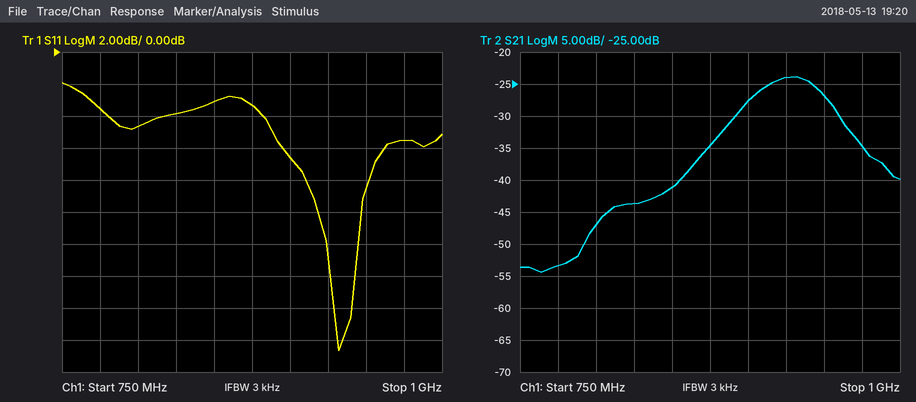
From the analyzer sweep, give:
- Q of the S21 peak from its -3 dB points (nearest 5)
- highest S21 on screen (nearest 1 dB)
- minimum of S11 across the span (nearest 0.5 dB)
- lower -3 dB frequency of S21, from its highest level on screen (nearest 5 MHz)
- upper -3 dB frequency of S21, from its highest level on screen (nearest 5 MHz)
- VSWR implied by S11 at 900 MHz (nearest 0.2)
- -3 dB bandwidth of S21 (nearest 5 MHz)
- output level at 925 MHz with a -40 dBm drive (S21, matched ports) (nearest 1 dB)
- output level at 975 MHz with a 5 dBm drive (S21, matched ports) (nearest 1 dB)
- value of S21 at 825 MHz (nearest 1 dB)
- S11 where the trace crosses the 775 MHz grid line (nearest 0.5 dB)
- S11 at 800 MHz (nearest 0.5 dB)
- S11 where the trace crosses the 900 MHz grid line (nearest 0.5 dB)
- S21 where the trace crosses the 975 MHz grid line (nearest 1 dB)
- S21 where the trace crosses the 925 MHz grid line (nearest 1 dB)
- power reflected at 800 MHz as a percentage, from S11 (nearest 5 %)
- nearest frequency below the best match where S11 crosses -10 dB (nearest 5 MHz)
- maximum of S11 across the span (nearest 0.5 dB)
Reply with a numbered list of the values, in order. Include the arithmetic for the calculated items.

1. 927.5 MHz / 45 MHz ≈ 20.6, so 20 to the nearest 5
2. -24 dB
3. -18.5 dB
4. 905 MHz
5. 950 MHz
6. |Γ| = 10^(-6.5/20) = 0.4732; VSWR = (1 + 0.4732)/(1 − 0.4732) ≈ 2.8
7. 950 MHz − 905 MHz = 45 MHz
8. -40 dBm + (-24 dB) = -64 dBm
9. 5 dBm + (-35 dB) = -30 dBm
10. -44 dB
11. -3.5 dB
12. -4.5 dB
13. -6.5 dB
14. -35 dB
15. -24 dB
16. 10^(-4.5/10) ≈ 35 %
17. 920 MHz
18. -2.0 dB
